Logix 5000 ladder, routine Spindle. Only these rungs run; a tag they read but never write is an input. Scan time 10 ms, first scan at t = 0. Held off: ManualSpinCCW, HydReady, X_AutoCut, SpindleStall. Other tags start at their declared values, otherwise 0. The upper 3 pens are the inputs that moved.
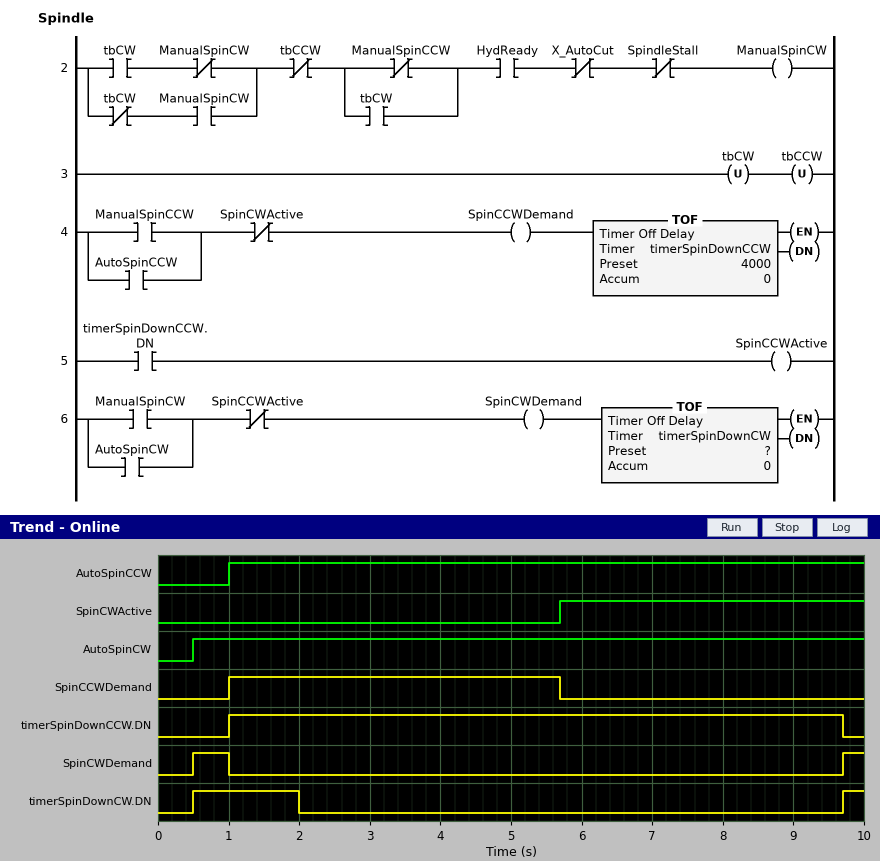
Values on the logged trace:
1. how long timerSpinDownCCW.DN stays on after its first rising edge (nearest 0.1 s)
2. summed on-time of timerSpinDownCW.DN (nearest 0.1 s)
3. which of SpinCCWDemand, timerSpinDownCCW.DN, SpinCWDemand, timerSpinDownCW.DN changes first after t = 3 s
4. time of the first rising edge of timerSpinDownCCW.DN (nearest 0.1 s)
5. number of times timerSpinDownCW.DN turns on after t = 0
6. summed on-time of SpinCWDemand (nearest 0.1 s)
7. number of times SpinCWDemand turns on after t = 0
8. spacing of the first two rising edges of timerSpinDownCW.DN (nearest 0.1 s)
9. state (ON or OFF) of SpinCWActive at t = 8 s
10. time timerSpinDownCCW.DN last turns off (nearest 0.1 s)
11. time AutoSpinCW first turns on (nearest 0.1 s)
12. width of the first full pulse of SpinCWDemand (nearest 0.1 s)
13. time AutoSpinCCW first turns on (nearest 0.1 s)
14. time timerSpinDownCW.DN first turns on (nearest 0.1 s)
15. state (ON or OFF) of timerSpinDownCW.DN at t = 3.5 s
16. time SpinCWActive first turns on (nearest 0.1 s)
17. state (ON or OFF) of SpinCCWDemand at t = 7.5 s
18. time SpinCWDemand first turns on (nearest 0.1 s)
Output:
8.7 s
1.8 s
SpinCCWDemand
1.0 s
2
0.8 s
2
9.2 s
ON
9.7 s
0.5 s
0.5 s
1.0 s
0.5 s
OFF
5.7 s
OFF
0.5 s
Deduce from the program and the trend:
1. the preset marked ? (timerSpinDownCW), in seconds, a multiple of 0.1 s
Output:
1.0 s
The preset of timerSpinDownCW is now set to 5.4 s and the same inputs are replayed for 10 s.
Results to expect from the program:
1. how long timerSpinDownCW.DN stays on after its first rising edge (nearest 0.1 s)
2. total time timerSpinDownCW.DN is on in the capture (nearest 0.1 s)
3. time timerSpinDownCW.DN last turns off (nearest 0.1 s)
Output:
5.9 s
6.2 s
6.4 s
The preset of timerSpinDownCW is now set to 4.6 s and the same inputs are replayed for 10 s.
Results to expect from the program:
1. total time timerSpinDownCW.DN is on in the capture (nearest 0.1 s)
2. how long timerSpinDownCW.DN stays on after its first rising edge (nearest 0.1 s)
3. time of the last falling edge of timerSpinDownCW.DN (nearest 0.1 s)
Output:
5.4 s
5.1 s
5.6 s
